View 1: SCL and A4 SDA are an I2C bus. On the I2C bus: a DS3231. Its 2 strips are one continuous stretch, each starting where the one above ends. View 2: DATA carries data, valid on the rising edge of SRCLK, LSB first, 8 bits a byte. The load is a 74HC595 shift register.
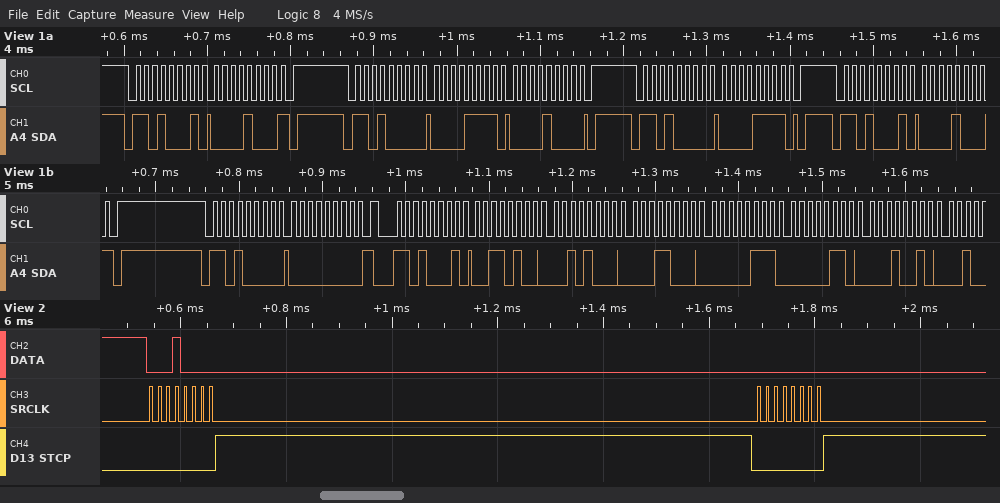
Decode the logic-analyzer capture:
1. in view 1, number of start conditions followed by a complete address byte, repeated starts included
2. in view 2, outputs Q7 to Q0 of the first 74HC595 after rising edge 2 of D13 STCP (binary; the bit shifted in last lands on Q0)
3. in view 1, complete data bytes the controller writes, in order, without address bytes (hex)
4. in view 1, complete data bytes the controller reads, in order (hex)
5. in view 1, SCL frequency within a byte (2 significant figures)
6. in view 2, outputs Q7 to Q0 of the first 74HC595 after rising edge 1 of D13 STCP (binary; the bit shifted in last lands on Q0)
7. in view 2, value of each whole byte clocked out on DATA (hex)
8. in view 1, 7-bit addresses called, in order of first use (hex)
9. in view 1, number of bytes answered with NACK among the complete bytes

6
00000000
0F 08 0F 00
08 08 34 28 18 07 06 12
100 kHz
00010000
08 00
0x68
2
